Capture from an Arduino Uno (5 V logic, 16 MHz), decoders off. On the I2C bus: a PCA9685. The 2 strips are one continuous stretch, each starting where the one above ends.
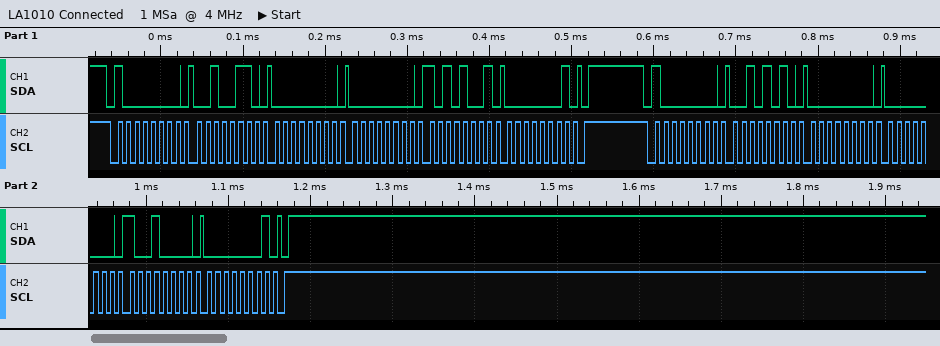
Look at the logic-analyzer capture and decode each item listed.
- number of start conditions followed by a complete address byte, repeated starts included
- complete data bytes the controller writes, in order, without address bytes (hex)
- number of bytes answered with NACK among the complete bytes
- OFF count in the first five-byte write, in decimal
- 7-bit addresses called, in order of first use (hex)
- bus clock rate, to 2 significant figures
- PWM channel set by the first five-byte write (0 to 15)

2
26 00 00 A9 01 2A 00 00 90 01
0
425
0x40
100 kHz
8
